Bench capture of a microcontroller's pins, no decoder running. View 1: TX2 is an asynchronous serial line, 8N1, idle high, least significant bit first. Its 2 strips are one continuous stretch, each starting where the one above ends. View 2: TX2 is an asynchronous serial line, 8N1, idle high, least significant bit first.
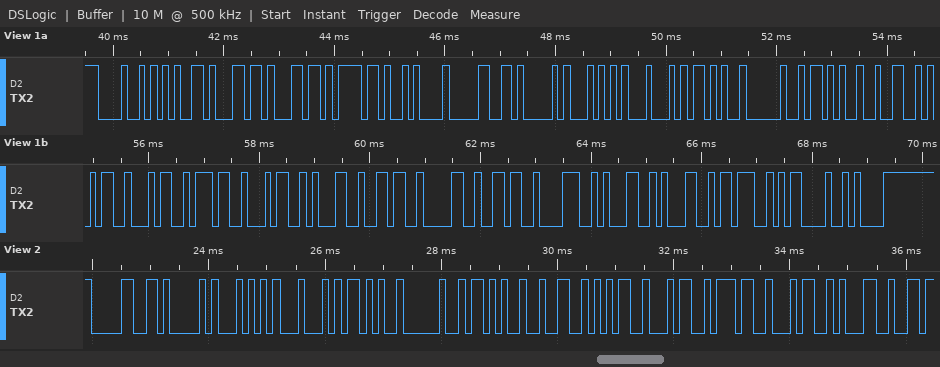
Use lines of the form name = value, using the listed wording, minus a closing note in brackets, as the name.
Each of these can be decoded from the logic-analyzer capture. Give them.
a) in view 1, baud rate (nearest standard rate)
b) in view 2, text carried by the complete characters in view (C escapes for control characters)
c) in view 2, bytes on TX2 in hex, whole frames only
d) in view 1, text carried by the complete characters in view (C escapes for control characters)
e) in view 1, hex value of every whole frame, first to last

in view 1, baud rate = 9600 baud
in view 2, text carried by the complete characters in view = "0ATD+ +254741"
in view 2, bytes on TX2 in hex, whole frames only = 30 41 54 44 2B 20 2B 32 35 34 37 34 31
in view 1, text carried by the complete characters in view = "Hello\n0ATD+ +254741606811;\r\n"
in view 1, hex value of every whole frame, first to last = 48 65 6C 6C 6F 0A 30 41 54 44 2B 20 2B 32 35 34 37 34 31 36 30 36 38 31 31 3B 0D 0A
